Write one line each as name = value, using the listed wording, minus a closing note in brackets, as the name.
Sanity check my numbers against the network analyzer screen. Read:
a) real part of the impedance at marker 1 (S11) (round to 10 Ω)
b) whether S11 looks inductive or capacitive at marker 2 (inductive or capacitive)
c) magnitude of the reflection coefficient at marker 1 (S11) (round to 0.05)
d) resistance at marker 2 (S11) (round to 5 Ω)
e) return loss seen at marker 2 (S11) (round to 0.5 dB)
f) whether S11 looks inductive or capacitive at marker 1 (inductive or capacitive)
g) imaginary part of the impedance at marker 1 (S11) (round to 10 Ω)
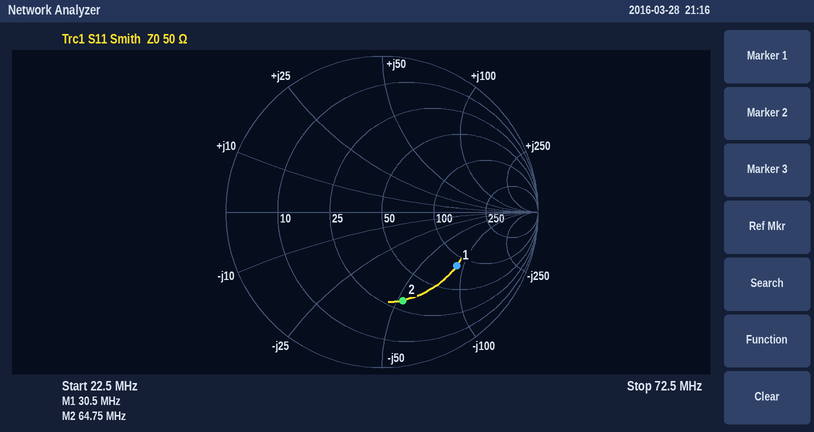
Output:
real part of the impedance at marker 1 (S11) = 80 Ω
whether S11 looks inductive or capacitive at marker 2 = capacitive
magnitude of the reflection coefficient at marker 1 (S11) = 0.60
resistance at marker 2 (S11) = 30 Ω
return loss seen at marker 2 (S11) = 4.5 dB
whether S11 looks inductive or capacitive at marker 1 = capacitive
imaginary part of the impedance at marker 1 (S11) = -90 Ω
